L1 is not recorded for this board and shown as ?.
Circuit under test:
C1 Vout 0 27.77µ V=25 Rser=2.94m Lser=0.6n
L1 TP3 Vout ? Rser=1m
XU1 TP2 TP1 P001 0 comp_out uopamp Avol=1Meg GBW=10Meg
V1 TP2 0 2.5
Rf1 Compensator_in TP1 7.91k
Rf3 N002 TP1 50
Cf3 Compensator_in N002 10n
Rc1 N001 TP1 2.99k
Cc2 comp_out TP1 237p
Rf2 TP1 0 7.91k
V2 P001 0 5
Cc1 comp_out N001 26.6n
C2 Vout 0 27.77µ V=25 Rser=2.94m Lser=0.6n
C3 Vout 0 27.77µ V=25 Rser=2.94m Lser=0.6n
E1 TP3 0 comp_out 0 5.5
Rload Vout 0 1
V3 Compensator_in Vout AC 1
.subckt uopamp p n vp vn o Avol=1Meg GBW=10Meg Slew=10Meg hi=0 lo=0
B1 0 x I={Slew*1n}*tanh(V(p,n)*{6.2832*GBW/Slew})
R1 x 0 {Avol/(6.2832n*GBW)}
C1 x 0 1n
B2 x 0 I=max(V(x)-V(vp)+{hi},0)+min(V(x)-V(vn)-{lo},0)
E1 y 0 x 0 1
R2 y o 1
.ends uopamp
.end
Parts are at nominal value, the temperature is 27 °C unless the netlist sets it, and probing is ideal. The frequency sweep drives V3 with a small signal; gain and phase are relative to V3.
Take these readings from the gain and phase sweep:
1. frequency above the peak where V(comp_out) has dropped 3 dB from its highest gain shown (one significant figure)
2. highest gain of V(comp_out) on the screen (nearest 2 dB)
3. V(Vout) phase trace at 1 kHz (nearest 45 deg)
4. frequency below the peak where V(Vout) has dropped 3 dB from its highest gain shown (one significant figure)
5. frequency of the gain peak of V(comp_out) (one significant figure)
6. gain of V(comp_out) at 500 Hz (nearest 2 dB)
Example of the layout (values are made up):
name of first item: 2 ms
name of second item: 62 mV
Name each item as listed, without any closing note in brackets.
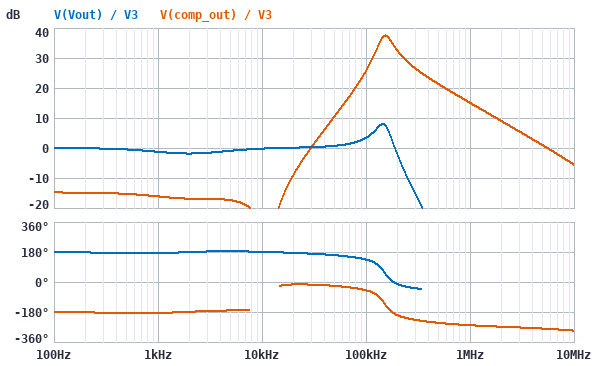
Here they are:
frequency above the peak where V(comp_out) has dropped 3 dB from its highest gain shown: 200 kHz
highest gain of V(comp_out) on the screen: 38 dB
V(Vout) phase trace at 1 kHz: 180 deg
frequency below the peak where V(Vout) has dropped 3 dB from its highest gain shown: 100 kHz
frequency of the gain peak of V(comp_out): 200 kHz
gain of V(comp_out) at 500 Hz: -16 dB
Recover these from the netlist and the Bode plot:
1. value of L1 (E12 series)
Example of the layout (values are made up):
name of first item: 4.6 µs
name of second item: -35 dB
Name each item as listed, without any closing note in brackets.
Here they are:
value of L1: 2.2 µH
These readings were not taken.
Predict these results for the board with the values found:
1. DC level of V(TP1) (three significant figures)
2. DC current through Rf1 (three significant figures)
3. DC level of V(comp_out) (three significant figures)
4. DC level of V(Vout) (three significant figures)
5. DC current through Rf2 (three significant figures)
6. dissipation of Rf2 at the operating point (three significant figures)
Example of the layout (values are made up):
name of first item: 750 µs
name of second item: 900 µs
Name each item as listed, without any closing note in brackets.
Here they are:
DC level of V(TP1): 2.50 V
DC current through Rf1: 316 µA
DC level of V(comp_out): 910 mV
DC level of V(Vout): 5.00 V
DC current through Rf2: 316 µA
dissipation of Rf2 at the operating point: 790 µW
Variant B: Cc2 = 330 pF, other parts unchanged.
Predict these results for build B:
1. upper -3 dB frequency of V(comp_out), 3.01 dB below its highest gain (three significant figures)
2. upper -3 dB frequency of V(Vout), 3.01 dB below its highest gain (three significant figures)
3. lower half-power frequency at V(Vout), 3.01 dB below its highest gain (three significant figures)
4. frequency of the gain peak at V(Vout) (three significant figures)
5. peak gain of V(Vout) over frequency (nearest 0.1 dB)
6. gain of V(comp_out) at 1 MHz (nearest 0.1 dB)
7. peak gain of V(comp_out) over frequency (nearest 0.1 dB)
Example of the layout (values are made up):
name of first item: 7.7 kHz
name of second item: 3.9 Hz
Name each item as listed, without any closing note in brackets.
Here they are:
upper -3 dB frequency of V(comp_out), 3.01 dB below its highest gain: 166 kHz
upper -3 dB frequency of V(Vout), 3.01 dB below its highest gain: 150 kHz
lower half-power frequency at V(Vout), 3.01 dB below its highest gain: 103 kHz
frequency of the gain peak at V(Vout): 130 kHz
peak gain of V(Vout) over frequency: 8.2 dB
gain of V(comp_out) at 1 MHz: 13.7 dB
peak gain of V(comp_out) over frequency: 35.7 dB
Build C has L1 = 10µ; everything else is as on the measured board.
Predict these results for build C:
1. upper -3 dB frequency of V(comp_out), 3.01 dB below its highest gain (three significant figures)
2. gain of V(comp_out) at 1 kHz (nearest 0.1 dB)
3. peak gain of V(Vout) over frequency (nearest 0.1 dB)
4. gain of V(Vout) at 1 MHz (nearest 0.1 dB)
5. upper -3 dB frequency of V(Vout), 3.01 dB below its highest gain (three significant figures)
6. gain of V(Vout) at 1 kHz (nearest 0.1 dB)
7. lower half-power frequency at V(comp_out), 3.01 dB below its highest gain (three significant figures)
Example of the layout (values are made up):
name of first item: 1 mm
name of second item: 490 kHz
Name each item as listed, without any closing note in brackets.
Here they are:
upper -3 dB frequency of V(comp_out), 3.01 dB below its highest gain: 281 kHz
gain of V(comp_out) at 1 kHz: -16.3 dB
peak gain of V(Vout) over frequency: 0.2 dB
gain of V(Vout) at 1 MHz: -64.8 dB
upper -3 dB frequency of V(Vout), 3.01 dB below its highest gain: 44.6 kHz
gain of V(Vout) at 1 kHz: -1.2 dB
lower half-power frequency at V(comp_out), 3.01 dB below its highest gain: 87.7 kHz
